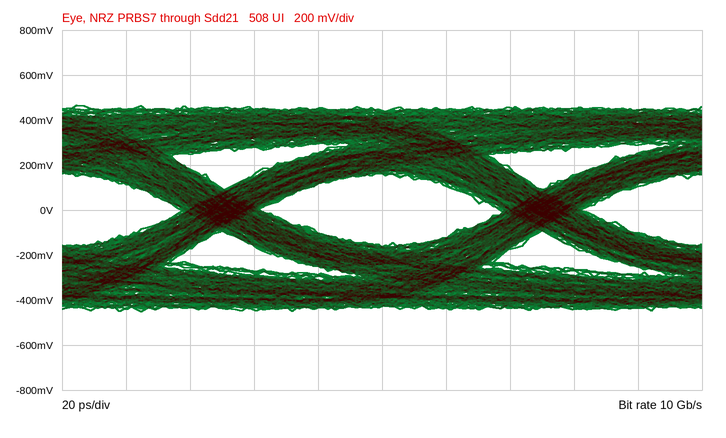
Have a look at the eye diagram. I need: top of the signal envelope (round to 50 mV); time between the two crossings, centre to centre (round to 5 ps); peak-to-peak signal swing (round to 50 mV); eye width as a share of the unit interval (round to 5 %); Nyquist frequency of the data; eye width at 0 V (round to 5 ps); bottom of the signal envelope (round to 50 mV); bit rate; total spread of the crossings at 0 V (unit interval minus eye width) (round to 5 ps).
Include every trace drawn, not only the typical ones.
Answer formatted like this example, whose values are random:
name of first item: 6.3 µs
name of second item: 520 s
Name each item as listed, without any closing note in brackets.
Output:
top of the signal envelope: 450 mV
time between the two crossings, centre to centre: 100 ps
peak-to-peak signal swing: 900 mV
eye width as a share of the unit interval: 75 %
Nyquist frequency of the data: 5 GHz
eye width at 0 V: 75 ps
bottom of the signal envelope: -450 mV
bit rate: 10 Gb/s
total spread of the crossings at 0 V (unit interval minus eye width): 25 ps
